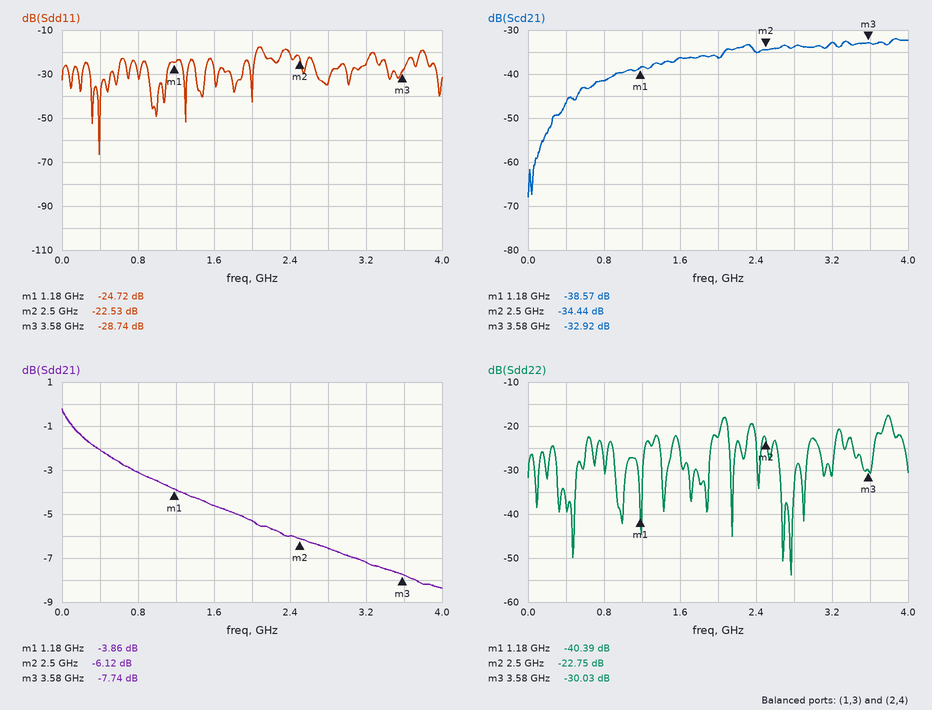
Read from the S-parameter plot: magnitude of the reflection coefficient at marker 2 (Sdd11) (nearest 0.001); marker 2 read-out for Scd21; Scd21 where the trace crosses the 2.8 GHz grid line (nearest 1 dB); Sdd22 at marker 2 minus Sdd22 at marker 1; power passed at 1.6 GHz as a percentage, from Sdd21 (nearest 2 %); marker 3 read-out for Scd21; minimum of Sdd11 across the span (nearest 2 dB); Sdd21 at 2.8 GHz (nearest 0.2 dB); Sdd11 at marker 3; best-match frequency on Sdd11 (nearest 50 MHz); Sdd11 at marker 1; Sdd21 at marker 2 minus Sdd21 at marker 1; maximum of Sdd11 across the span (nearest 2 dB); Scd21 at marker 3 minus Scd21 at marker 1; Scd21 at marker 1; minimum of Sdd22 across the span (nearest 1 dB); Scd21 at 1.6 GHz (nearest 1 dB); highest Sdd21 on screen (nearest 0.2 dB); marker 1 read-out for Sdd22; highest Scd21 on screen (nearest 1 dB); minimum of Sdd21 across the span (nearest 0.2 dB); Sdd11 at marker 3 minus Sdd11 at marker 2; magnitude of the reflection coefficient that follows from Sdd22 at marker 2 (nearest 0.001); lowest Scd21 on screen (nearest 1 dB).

0.075
-34.44 dB
-34 dB
17.64 dB
34 %
-32.92 dB
-66 dB
-6.6 dB
-28.74 dB
400 MHz
-24.72 dB
-2.26 dB
-18 dB
5.65 dB
-38.57 dB
-54 dB
-36 dB
-0.2 dB
-40.39 dB
-32 dB
-8.4 dB
-6.21 dB
0.073
-68 dB
